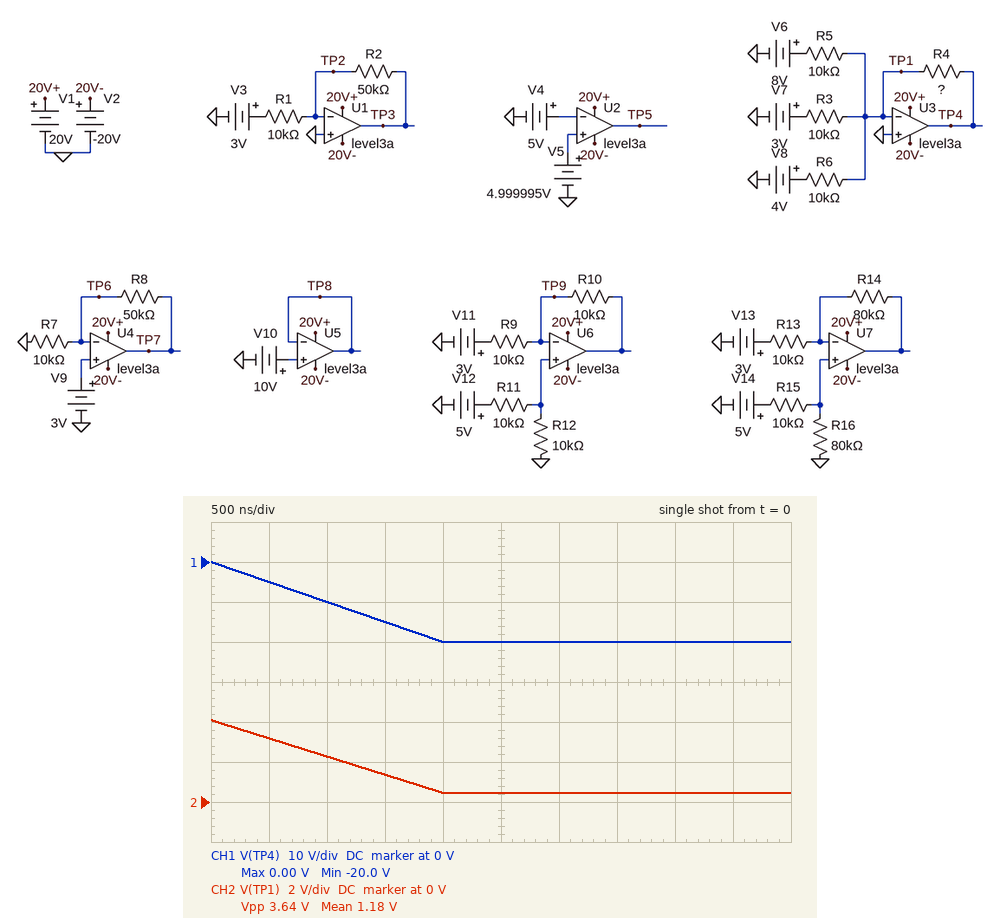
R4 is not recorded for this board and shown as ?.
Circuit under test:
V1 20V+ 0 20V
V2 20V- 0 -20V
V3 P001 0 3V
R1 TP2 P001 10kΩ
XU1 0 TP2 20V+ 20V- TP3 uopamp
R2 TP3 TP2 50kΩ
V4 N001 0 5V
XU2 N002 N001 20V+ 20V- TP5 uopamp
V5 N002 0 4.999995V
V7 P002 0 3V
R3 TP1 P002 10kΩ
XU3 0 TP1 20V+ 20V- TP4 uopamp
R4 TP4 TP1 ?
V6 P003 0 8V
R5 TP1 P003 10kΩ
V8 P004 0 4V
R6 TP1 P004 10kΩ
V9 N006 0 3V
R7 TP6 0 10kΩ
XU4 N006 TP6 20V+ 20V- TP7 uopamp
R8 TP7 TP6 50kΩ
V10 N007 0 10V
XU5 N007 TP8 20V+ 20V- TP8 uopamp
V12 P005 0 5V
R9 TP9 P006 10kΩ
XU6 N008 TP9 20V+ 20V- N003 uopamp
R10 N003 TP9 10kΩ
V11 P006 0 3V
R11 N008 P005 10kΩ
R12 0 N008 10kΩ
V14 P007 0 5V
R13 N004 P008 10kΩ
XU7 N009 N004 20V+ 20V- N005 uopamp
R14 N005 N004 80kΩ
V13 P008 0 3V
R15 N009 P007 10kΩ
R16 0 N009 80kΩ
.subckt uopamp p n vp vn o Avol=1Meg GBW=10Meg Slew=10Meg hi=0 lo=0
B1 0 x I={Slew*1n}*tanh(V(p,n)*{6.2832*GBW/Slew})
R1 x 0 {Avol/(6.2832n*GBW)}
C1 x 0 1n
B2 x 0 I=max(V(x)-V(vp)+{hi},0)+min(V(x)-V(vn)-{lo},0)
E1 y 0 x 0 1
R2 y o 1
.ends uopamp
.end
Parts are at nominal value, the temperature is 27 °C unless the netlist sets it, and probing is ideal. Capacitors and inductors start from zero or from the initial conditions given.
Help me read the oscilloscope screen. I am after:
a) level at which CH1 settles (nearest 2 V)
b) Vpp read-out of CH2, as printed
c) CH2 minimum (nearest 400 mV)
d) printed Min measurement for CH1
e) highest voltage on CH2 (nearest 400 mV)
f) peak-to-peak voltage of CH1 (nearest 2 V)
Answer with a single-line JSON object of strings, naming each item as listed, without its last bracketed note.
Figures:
{"level at which CH1 settles": "-20 V", "Vpp read-out of CH2, as printed": "3.64 V", "CH2 minimum": "400 mV", "printed Min measurement for CH1": "-20.0 V", "highest voltage on CH2": "4.0 V", "peak-to-peak voltage of CH1": "20 V"}
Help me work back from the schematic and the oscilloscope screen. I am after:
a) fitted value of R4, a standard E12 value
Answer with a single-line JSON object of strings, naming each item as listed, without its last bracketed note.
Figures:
{"fitted value of R4, a standard E12 value": "15 kΩ"}
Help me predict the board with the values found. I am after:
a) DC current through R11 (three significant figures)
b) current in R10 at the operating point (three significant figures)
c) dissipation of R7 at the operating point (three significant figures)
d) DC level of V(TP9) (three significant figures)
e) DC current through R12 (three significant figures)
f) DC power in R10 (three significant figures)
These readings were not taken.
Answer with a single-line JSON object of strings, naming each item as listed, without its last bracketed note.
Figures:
{"DC current through R11": "250 µA", "current in R10 at the operating point": "50.0 µA", "dissipation of R7 at the operating point": "900 µW", "DC level of V(TP9)": "2.50 V", "DC current through R12": "250 µA", "DC power in R10": "25.0 µW"}
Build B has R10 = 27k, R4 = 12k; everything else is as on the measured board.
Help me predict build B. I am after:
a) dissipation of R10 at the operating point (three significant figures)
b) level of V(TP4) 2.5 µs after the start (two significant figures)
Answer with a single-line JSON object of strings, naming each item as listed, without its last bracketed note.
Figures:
{"dissipation of R10 at the operating point": "67.5 µW", "level of V(TP4) 2.5 µs after the start": "-18 V"}
